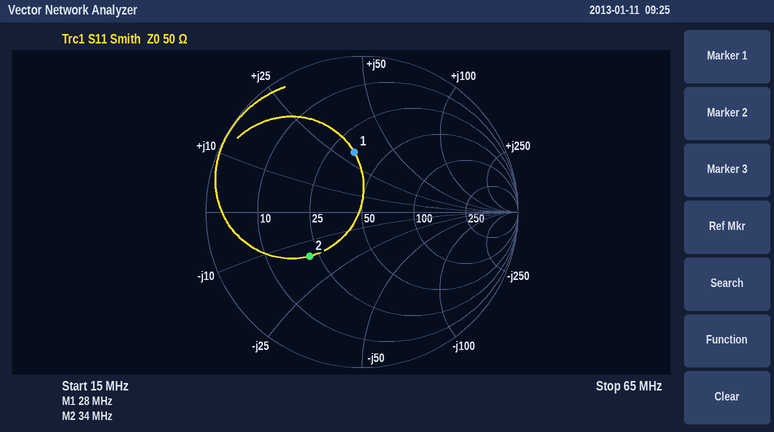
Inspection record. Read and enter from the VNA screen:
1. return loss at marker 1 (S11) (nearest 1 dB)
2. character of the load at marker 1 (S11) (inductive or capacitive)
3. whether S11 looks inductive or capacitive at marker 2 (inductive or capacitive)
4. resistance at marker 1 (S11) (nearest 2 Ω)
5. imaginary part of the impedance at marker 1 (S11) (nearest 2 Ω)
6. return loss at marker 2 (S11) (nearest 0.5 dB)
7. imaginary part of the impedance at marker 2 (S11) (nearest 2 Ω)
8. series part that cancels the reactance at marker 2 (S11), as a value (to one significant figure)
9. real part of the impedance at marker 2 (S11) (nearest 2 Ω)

8 dB
inductive
capacitive
34 Ω
+30 Ω
7.0 dB
-16 Ω
70 nH
22 Ω
